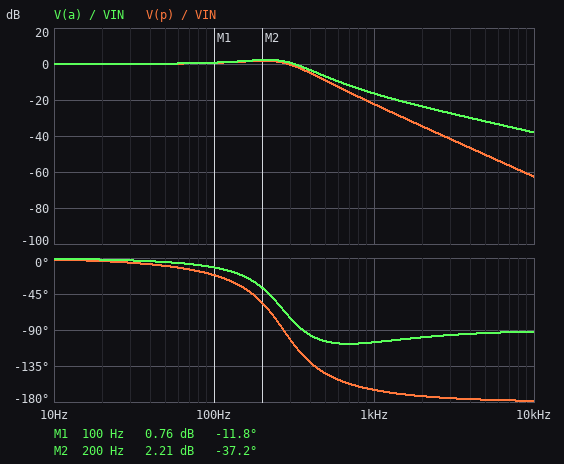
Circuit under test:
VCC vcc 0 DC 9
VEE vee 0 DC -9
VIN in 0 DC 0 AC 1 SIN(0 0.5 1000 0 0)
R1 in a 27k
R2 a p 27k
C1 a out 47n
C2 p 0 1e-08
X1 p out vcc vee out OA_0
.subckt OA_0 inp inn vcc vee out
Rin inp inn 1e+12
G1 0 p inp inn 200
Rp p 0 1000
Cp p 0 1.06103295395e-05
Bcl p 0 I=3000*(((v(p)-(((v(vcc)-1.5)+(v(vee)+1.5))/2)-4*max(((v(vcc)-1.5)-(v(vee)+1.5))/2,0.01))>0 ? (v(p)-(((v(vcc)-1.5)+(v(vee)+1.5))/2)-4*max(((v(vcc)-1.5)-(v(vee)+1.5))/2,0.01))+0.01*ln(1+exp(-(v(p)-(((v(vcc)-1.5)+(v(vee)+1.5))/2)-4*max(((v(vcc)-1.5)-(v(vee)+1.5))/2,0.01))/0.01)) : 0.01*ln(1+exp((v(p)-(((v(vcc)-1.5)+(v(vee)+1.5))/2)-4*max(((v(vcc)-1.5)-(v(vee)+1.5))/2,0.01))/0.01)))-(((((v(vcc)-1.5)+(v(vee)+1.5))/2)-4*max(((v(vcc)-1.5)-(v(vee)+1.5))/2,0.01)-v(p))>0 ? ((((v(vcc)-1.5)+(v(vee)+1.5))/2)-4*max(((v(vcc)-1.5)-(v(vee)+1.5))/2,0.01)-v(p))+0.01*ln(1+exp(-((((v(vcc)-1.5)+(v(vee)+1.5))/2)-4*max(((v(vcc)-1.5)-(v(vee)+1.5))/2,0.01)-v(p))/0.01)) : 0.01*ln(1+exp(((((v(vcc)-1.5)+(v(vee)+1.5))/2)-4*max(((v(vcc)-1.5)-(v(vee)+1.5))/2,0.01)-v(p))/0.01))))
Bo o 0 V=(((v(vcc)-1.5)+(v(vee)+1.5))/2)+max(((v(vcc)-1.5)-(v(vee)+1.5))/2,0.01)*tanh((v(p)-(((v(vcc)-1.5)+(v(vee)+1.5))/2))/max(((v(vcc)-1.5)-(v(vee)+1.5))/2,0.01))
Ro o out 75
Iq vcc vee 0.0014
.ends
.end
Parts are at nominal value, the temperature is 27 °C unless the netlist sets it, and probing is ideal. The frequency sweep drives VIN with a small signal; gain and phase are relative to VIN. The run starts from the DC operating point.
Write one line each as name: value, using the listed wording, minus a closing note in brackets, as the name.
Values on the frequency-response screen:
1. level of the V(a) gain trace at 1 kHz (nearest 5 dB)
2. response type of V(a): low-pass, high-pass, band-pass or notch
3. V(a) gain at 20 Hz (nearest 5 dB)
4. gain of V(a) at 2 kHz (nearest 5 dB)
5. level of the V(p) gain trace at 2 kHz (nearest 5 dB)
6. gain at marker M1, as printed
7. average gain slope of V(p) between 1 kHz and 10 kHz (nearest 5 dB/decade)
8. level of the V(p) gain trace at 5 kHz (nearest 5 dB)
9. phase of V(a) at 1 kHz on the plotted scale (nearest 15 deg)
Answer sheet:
level of the V(a) gain trace at 1 kHz: -15 dB
response type of V(a): low-pass, high-pass, band-pass or notch: low-pass
V(a) gain at 20 Hz: 0 dB
gain of V(a) at 2 kHz: -25 dB
level of the V(p) gain trace at 2 kHz: -35 dB
gain at marker M1, as printed: 0.76 dB
average gain slope of V(p) between 1 kHz and 10 kHz: -40 dB/decade
level of the V(p) gain trace at 5 kHz: -50 dB
phase of V(a) at 1 kHz on the plotted scale: -105 deg
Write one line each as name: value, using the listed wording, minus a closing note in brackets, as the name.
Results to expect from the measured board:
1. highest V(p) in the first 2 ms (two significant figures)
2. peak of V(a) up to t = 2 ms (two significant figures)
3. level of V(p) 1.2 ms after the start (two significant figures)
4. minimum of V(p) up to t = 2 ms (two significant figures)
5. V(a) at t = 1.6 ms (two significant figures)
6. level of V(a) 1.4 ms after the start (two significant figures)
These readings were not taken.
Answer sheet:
highest V(p) in the first 2 ms: 120 mV
peak of V(a) up to t = 2 ms: 170 mV
level of V(p) 1.2 ms after the start: 21 mV
minimum of V(p) up to t = 2 ms: -8.6 mV
V(a) at t = 1.6 ms: 78 mV
level of V(a) 1.4 ms after the start: 69 mV
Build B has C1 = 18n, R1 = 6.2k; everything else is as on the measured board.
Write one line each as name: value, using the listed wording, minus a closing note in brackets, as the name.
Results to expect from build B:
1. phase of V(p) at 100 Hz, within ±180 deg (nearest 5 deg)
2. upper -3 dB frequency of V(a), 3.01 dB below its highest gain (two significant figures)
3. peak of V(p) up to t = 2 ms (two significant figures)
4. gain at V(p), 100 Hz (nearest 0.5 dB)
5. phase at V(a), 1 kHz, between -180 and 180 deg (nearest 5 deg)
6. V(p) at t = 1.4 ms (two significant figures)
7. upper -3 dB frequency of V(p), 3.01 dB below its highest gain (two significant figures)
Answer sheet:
phase of V(p) at 100 Hz, within ±180 deg: -10 deg
upper -3 dB frequency of V(a), 3.01 dB below its highest gain: 1.6 kHz
peak of V(p) up to t = 2 ms: 290 mV
gain at V(p), 100 Hz: 0 dB
phase at V(a), 1 kHz, between -180 and 180 deg: -35 deg
V(p) at t = 1.4 ms: 180 mV
upper -3 dB frequency of V(p), 3.01 dB below its highest gain: 630 Hz
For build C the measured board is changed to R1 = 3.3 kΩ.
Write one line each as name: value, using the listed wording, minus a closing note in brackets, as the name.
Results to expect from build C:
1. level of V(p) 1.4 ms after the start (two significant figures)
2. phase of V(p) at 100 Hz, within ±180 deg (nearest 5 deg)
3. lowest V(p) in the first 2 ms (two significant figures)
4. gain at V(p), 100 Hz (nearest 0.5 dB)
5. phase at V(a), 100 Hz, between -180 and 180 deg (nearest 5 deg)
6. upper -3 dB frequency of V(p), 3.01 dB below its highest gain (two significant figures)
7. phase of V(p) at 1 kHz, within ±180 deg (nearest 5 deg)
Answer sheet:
level of V(p) 1.4 ms after the start: 140 mV
phase of V(p) at 100 Hz, within ±180 deg: -10 deg
lowest V(p) in the first 2 ms: -260 mV
gain at V(p), 100 Hz: 0 dB
phase at V(a), 100 Hz, between -180 and 180 deg: 0 deg
upper -3 dB frequency of V(p), 3.01 dB below its highest gain: 740 Hz
phase of V(p) at 1 kHz, within ±180 deg: -110 deg
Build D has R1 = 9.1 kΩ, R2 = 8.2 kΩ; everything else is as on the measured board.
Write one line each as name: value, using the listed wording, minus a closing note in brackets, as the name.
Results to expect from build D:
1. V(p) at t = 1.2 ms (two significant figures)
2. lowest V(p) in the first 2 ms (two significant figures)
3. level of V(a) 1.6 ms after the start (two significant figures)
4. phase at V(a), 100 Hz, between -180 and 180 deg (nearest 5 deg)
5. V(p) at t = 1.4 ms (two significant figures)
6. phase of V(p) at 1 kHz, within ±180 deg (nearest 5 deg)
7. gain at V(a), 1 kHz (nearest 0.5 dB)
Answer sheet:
V(p) at t = 1.2 ms: -260 mV
lowest V(p) in the first 2 ms: -460 mV
level of V(a) 1.6 ms after the start: 360 mV
phase at V(a), 100 Hz, between -180 and 180 deg: -5 deg
V(p) at t = 1.4 ms: 260 mV
phase of V(p) at 1 kHz, within ±180 deg: -110 deg
gain at V(a), 1 kHz: 0 dB
